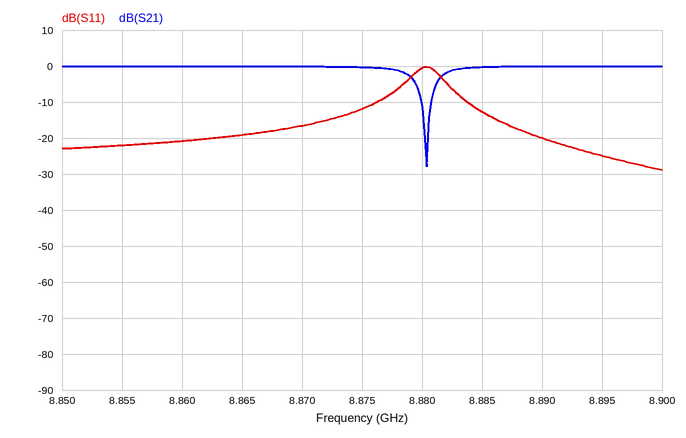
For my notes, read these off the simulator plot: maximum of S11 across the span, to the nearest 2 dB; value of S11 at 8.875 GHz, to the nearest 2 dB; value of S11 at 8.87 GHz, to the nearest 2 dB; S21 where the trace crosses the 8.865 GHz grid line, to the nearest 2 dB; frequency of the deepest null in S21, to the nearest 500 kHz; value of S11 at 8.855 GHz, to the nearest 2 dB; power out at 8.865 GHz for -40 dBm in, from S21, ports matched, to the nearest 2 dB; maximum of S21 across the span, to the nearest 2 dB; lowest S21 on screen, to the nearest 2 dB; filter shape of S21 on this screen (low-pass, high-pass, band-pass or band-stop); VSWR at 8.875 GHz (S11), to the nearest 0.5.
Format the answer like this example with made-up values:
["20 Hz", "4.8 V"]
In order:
["0 dB", "-12 dB", "-16 dB", "0 dB", "8.8805 GHz", "-22 dB", "-40 dBm", "0 dB", "-28 dB", "band-stop", "1.5"]
